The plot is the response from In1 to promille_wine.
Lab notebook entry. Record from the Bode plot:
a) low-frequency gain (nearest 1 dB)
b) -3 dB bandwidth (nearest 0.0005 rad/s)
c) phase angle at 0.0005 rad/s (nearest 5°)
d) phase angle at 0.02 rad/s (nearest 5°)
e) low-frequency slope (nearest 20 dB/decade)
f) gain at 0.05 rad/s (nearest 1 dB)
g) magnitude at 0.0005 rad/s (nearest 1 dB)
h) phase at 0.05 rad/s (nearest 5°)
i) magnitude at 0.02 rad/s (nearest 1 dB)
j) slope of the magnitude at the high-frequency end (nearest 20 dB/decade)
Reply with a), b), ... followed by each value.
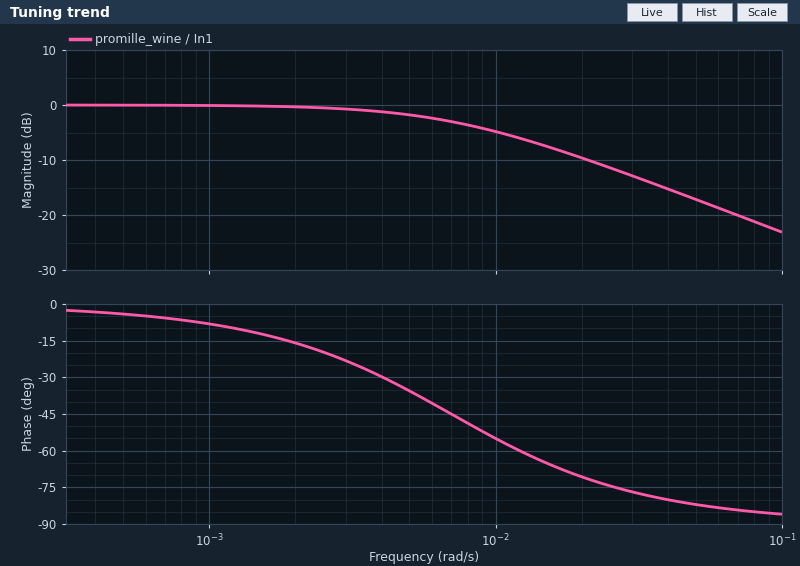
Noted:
a) 0 dB
b) 0.0070 rad/s
c) -5°
d) -70°
e) 0 dB/decade
f) -17 dB
g) 0 dB
h) -80°
i) -10 dB
j) -20 dB/decade
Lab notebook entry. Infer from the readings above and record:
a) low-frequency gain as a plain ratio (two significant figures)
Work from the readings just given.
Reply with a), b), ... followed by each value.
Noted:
a) 1.0
